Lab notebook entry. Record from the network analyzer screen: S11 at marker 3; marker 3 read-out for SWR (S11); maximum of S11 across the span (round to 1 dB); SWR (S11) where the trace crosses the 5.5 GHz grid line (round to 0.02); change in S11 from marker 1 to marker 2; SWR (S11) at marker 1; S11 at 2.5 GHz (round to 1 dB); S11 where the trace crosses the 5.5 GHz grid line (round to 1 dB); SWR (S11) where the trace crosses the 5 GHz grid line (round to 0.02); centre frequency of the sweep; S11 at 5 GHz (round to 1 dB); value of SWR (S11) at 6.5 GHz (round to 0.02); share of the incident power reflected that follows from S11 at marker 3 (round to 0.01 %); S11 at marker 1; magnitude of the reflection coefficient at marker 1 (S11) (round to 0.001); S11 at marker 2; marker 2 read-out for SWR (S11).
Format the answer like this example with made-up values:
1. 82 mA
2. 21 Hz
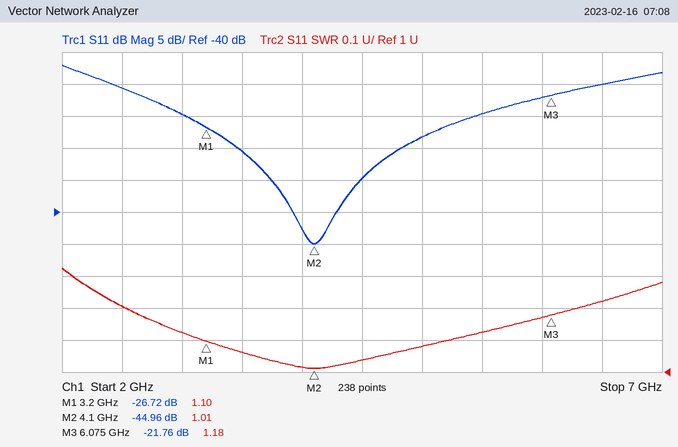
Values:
1. -21.76 dB
2. 1.18
3. -17 dB
4. 1.12
5. -18.24 dB
6. 1.10
7. -21 dB
8. -25 dB
9. 1.08
10. 4.5 GHz
11. -28 dB
12. 1.22
13. 0.67 %
14. -26.72 dB
15. 0.046
16. -44.96 dB
17. 1.01
